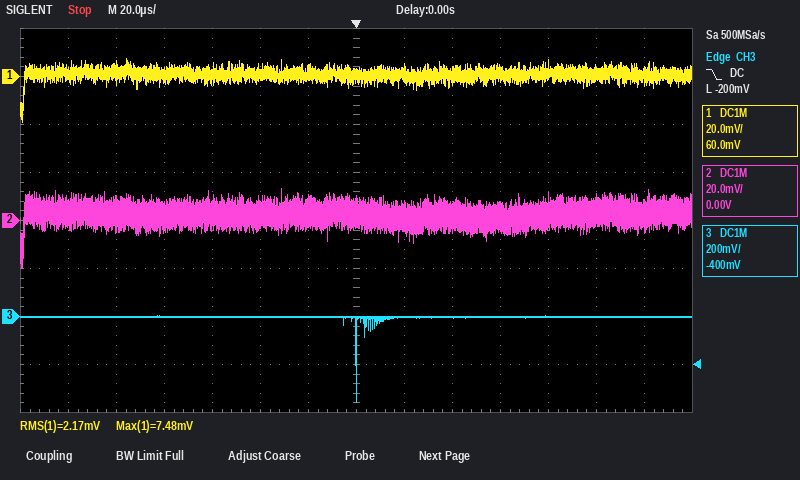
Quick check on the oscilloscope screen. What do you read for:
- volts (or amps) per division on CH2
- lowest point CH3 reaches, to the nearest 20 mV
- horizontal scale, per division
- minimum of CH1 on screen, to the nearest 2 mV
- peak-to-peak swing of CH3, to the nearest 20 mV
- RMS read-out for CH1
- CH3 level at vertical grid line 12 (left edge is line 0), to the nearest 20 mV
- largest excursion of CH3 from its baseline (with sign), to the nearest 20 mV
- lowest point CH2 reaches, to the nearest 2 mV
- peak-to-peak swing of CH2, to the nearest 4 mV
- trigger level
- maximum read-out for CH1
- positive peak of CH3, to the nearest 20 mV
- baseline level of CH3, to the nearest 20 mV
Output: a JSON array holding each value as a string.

["20 mV", "-360 mV", "20 µs", "-18 mV", "360 mV", "2.17 mV", "0 mV", "-360 mV", "-20 mV", "32 mV", "-200 mV", "7.48 mV", "0 mV", "0 mV"]
